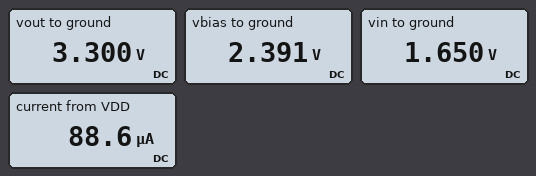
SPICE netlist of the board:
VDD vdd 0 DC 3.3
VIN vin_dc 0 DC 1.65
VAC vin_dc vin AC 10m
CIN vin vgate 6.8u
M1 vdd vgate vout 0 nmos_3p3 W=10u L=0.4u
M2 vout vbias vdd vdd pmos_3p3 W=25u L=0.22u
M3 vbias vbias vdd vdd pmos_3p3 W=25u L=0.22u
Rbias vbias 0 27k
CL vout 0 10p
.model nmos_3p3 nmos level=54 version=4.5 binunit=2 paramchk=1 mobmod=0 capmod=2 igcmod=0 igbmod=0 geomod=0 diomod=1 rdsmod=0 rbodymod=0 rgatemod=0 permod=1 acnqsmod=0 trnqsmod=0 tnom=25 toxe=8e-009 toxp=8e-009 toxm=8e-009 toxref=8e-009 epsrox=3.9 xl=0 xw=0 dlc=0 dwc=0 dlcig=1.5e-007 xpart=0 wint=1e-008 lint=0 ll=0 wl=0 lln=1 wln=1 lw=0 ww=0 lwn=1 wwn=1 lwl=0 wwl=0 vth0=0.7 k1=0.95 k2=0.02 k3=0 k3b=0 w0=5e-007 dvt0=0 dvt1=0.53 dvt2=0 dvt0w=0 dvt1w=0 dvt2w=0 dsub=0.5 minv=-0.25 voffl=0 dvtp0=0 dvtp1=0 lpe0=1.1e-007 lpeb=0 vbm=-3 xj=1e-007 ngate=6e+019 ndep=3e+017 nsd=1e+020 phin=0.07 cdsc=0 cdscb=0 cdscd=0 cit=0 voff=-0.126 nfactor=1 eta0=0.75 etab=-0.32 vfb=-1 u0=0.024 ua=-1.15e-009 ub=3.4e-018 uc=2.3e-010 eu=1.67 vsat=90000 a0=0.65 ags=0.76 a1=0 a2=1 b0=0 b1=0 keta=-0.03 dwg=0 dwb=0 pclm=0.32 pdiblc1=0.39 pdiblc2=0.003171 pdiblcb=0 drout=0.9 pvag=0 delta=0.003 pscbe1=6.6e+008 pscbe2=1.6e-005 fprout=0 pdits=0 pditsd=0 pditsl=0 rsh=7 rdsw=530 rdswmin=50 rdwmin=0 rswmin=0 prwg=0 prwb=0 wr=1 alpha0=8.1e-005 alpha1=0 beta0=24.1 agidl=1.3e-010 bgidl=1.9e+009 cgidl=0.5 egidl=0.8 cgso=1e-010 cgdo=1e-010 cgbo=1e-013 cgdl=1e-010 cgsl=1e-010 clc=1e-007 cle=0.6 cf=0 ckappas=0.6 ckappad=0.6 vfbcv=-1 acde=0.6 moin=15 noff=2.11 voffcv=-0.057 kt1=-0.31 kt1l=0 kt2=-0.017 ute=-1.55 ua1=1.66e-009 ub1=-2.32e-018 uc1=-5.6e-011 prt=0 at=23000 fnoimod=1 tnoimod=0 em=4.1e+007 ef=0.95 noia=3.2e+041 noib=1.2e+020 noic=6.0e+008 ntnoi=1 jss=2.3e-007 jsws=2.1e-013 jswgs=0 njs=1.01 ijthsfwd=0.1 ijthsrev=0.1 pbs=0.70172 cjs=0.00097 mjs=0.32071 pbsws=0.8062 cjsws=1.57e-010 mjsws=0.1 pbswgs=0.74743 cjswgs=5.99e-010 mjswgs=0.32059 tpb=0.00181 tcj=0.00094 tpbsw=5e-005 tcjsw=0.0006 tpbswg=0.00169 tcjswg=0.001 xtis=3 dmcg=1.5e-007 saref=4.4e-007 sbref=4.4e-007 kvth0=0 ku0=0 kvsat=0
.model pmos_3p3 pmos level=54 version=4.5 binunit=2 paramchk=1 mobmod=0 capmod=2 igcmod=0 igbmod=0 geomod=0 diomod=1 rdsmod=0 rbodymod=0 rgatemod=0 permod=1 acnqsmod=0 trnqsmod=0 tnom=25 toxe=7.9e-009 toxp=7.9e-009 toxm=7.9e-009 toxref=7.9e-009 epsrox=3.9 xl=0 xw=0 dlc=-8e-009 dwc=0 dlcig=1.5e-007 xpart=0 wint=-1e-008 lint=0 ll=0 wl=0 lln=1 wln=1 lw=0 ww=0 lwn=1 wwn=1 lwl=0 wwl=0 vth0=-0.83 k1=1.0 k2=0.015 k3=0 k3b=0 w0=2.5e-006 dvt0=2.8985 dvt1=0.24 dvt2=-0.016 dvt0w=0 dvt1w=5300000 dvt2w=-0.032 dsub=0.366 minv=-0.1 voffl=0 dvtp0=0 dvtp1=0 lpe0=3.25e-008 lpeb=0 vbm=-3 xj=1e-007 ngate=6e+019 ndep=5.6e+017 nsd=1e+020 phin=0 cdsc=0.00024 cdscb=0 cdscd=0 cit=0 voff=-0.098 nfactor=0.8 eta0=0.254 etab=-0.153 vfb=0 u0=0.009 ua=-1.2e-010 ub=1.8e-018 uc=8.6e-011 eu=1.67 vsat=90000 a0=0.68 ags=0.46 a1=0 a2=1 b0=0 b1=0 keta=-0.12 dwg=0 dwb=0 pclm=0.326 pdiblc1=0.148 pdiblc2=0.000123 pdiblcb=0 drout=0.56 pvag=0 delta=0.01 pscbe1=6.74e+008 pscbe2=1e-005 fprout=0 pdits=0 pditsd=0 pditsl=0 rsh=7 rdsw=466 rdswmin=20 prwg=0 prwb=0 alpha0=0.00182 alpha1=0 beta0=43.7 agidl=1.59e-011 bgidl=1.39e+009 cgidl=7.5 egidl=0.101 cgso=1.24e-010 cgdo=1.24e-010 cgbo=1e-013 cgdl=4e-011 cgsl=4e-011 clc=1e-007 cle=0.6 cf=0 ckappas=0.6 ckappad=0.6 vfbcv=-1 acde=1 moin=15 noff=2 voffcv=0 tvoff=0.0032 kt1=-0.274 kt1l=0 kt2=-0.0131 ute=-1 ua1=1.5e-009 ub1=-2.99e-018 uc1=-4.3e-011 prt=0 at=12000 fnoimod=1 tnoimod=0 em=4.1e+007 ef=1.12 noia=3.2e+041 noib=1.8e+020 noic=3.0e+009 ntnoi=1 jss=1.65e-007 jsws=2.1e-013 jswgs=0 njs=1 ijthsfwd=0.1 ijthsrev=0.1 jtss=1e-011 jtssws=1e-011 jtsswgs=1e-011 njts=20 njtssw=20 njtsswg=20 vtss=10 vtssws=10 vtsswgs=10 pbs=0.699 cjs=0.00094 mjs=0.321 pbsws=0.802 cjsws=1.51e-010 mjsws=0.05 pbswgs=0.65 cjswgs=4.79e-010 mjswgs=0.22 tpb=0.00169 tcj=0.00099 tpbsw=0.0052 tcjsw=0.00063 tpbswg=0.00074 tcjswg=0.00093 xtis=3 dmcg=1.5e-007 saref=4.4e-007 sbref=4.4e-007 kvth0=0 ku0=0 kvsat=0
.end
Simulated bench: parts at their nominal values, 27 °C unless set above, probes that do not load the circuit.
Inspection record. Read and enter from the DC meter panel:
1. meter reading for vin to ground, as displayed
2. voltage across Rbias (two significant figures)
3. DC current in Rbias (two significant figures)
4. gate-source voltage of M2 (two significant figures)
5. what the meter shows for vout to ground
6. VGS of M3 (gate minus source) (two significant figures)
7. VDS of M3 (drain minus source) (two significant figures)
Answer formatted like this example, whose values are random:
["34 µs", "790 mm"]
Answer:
["1.650 V", "2.4 V", "89 µA", "-910 mV", "3.300 V", "-910 mV", "-910 mV"]
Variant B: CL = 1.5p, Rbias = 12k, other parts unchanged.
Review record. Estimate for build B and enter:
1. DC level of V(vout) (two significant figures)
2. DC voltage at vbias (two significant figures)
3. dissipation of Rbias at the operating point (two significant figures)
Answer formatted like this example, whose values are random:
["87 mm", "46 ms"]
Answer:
["3.3 V", "2.3 V", "430 µW"]
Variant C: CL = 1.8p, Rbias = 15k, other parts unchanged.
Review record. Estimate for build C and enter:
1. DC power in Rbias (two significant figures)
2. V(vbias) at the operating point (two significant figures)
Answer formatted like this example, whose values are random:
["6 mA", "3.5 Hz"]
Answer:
["360 µW", "2.3 V"]
